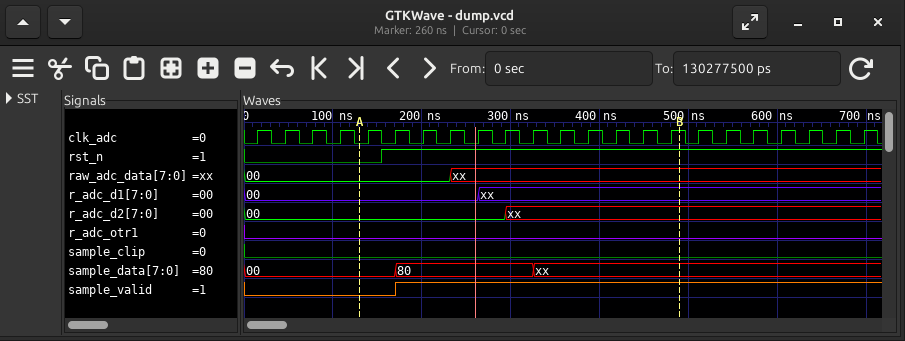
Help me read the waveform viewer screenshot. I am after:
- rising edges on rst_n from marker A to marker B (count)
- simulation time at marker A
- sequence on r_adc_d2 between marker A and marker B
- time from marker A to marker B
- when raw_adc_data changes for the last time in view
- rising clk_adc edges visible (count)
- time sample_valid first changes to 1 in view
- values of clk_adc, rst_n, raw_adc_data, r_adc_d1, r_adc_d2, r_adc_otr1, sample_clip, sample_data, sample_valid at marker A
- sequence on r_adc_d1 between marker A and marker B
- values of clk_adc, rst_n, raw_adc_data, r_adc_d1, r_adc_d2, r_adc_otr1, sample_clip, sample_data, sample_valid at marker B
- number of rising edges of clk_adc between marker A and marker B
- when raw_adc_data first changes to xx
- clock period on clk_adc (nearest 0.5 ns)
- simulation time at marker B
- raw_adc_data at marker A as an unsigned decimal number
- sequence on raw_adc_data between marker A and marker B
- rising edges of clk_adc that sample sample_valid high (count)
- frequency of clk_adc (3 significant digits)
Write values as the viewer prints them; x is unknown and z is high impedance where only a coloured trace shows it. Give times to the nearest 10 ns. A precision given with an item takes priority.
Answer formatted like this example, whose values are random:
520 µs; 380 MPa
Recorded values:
1; 130 ns; 00, xx; 360 ns; 230 ns; 23; 170 ns; clk_adc=0, rst_n=0, raw_adc_data=00, r_adc_d1=00, r_adc_d2=00, r_adc_otr1=0, sample_clip=0, sample_data=00, sample_valid=0; 00, xx; clk_adc=1, rst_n=1, raw_adc_data=xx, r_adc_d1=xx, r_adc_d2=xx, r_adc_otr1=0, sample_clip=0, sample_data=xx, sample_valid=1; 12; 230 ns; 31 ns; 490 ns; 0; 00, xx; 17; 32.3 MHz
